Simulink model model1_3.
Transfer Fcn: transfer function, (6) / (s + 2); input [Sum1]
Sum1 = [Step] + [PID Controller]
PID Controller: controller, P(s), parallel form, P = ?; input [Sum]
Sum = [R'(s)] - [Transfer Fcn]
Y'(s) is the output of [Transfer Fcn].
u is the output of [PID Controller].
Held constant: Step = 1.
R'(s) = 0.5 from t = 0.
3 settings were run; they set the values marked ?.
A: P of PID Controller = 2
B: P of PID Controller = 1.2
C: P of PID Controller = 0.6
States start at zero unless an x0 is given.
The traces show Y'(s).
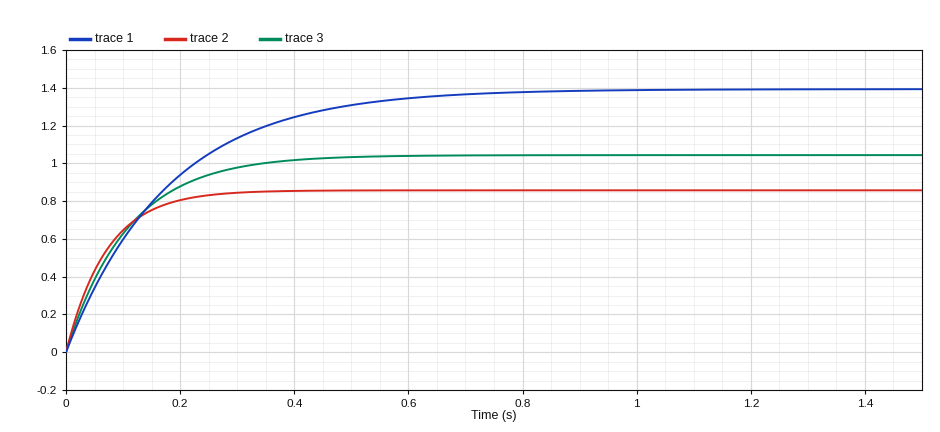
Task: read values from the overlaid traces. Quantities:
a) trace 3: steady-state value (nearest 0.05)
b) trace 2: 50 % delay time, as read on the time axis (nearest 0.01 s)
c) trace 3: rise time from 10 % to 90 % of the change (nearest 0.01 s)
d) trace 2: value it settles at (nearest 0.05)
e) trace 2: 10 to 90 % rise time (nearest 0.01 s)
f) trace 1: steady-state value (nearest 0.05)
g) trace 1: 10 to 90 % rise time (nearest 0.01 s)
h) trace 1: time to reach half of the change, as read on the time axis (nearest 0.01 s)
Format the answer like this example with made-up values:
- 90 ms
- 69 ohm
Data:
- 1.05
- 0.05 s
- 0.24 s
- 0.85
- 0.16 s
- 1.40
- 0.39 s
- 0.12 s
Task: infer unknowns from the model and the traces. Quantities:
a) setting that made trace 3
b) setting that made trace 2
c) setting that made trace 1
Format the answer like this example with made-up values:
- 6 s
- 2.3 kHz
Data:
- B
- A
- C
